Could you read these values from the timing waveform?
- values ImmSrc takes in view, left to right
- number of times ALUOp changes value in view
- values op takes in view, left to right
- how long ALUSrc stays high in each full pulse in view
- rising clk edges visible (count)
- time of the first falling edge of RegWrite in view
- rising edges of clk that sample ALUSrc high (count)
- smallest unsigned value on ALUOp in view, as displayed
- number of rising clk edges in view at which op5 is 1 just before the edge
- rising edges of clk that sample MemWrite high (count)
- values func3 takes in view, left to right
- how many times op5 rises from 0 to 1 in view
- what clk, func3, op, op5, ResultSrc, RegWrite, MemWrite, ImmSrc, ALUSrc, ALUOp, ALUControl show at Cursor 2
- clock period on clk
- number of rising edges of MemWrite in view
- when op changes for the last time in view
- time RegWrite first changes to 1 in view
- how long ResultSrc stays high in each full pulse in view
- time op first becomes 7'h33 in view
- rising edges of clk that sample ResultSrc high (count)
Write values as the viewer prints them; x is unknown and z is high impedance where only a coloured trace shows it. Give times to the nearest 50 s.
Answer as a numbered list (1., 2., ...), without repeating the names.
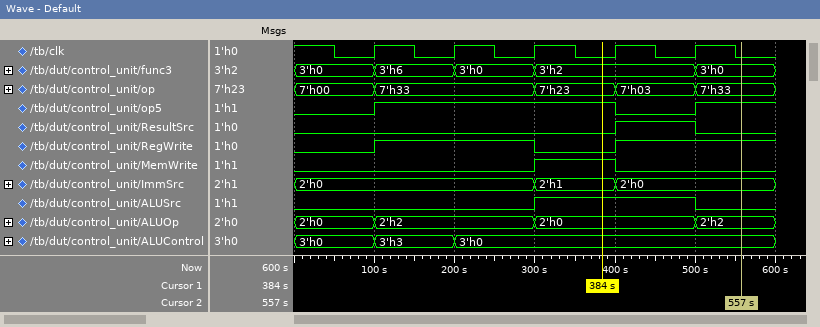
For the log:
1. 2'h0, 2'h1, 2'h0
2. 3
3. 7'h00, 7'h33, 7'h23, 7'h03, 7'h33
4. 200 s
5. 5
6. 300 s
7. 2
8. 2'h0
9. 3
10. 1
11. 3'h0, 3'h6, 3'h0, 3'h2, 3'h0
12. 2
13. clk=0, func3=3'h0, op=7'h33, op5=1, ResultSrc=0, RegWrite=1, MemWrite=0, ImmSrc=2'h0, ALUSrc=0, ALUOp=2'h2, ALUControl=3'h0
14. 100 s
15. 1
16. 500 s
17. 100 s
18. 100 s
19. 100 s
20. 1
